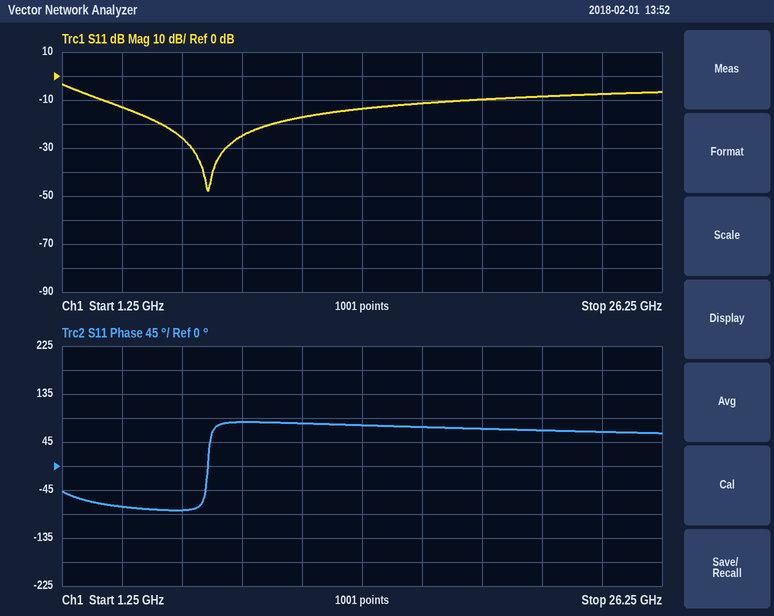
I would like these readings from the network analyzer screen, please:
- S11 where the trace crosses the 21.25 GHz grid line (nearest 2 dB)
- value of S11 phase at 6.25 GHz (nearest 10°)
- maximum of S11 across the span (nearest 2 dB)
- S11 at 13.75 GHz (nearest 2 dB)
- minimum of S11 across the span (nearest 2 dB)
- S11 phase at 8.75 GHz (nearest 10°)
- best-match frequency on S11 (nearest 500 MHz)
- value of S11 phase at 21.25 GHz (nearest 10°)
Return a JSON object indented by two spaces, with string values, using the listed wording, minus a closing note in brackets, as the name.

{
  "S11 where the trace crosses the 21.25 GHz grid line": "-8 dB",
  "value of S11 phase at 6.25 GHz": "-80°",
  "maximum of S11 across the span": "-4 dB",
  "S11 at 13.75 GHz": "-14 dB",
  "minimum of S11 across the span": "-48 dB",
  "S11 phase at 8.75 GHz": "80°",
  "best-match frequency on S11": "7.5 GHz",
  "value of S11 phase at 21.25 GHz": "70°"
}
